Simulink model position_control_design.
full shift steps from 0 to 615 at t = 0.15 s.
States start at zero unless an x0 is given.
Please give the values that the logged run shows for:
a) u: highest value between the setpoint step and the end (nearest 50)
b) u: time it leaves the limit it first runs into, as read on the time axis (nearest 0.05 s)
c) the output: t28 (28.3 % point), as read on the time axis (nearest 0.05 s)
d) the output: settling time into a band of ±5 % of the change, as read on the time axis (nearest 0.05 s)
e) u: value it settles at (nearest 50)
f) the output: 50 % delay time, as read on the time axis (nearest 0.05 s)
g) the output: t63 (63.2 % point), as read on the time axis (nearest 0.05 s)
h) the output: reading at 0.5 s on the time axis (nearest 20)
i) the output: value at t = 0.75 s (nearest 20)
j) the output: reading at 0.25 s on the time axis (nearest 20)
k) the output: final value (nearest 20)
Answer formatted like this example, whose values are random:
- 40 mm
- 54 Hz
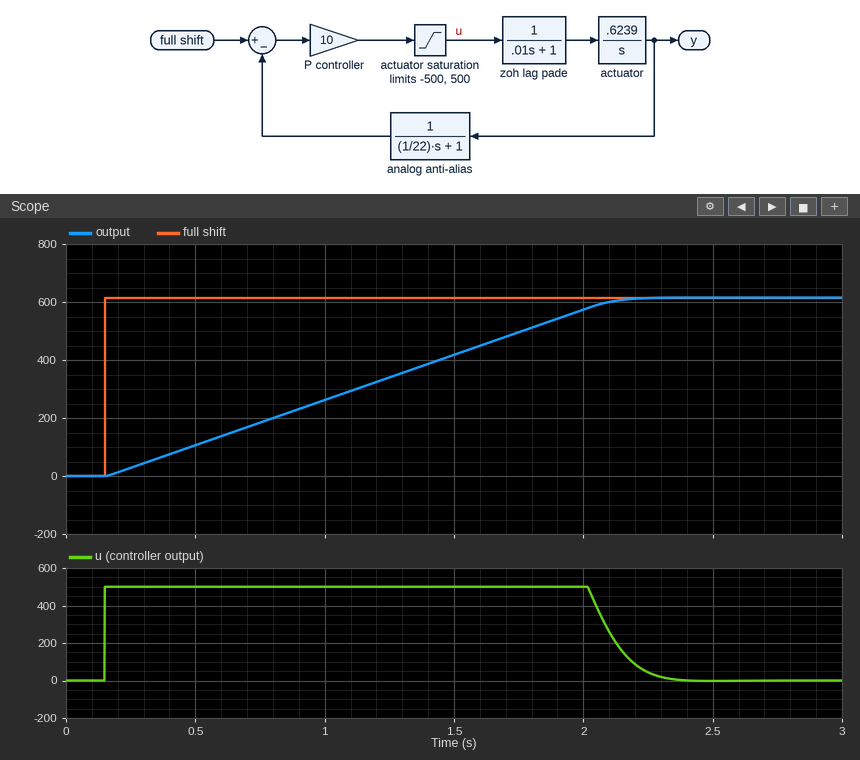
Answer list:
- 500
- 2.00 s
- 0.70 s
- 2.05 s
- 0
- 1.15 s
- 1.40 s
- 100
- 180
- 20
- 620
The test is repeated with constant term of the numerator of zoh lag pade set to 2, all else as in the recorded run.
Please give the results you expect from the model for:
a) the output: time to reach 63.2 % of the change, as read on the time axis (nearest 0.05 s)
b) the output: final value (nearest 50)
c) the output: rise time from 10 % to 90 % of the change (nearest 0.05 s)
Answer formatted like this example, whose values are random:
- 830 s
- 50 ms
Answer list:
- 0.80 s
- 600
- 0.80 s
